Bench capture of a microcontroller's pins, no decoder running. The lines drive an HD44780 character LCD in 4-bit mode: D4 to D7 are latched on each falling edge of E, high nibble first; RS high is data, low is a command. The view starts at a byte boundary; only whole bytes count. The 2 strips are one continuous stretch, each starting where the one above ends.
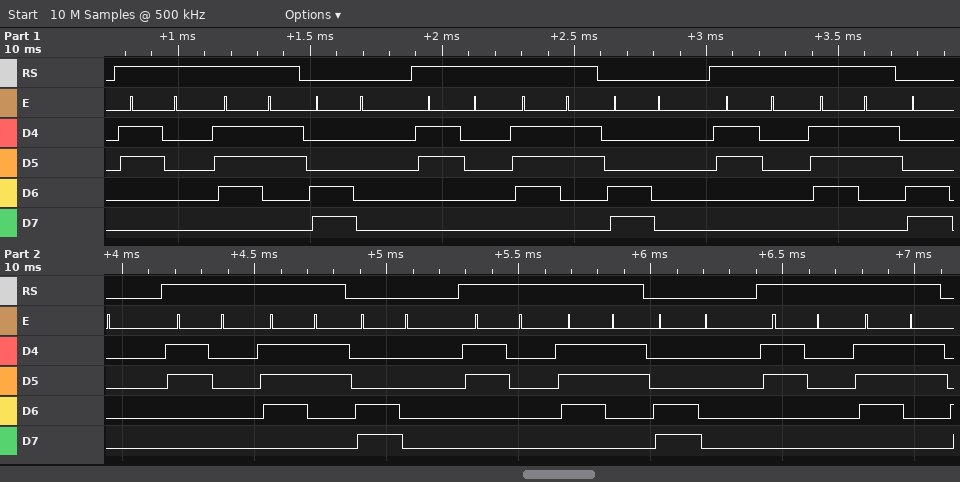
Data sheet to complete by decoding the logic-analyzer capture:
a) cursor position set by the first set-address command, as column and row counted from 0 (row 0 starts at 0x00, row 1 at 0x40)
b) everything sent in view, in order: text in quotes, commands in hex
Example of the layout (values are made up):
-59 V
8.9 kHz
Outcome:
column 0, row 1
"0s" 0xC0 "0s" 0xC0 "0s" 0xC0 "0s" 0xC0 "0s" 0xC0 "0s"
